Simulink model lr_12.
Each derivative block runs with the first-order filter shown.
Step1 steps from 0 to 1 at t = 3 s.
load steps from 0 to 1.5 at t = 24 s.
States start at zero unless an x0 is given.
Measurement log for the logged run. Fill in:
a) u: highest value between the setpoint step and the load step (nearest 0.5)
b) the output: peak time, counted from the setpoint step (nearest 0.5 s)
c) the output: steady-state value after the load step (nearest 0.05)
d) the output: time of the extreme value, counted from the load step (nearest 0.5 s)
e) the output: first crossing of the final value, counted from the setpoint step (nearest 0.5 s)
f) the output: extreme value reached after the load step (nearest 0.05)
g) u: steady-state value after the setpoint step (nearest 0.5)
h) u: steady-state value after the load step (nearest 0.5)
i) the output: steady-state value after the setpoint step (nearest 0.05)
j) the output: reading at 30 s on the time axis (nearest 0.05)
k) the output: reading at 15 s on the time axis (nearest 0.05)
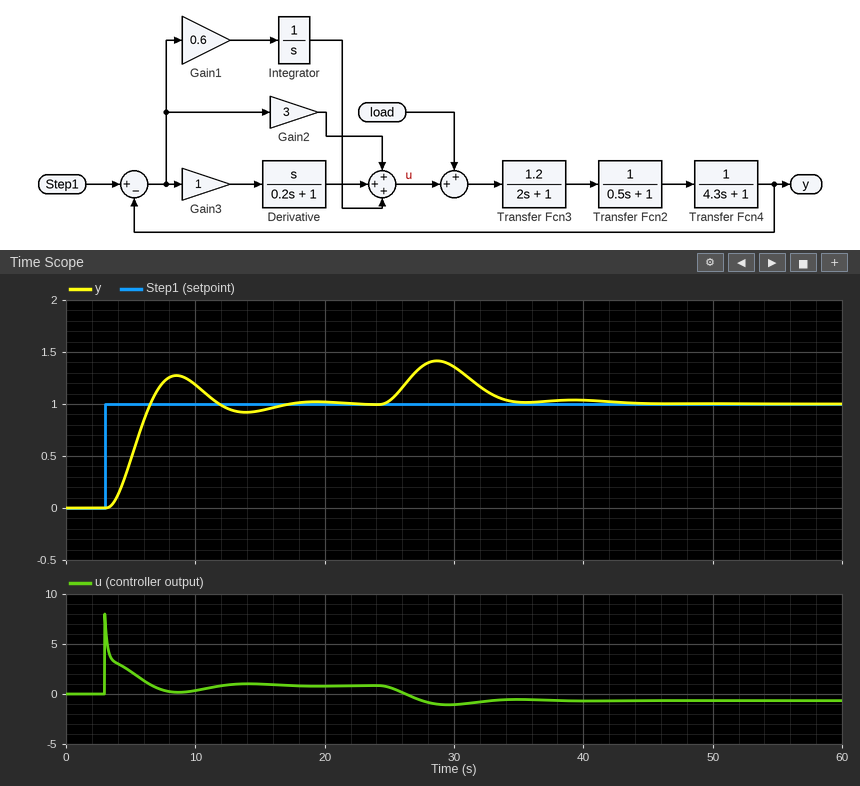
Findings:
8.0
5.5 s
1.00
4.5 s
3.5 s
1.40
1.0
-0.5
1.00
1.35
0.95
